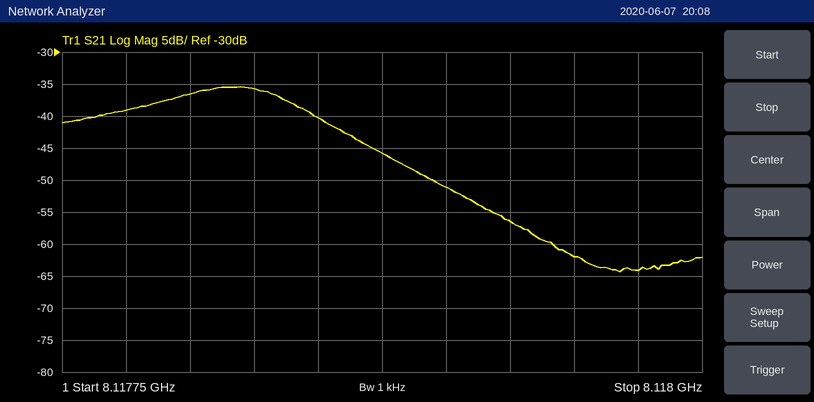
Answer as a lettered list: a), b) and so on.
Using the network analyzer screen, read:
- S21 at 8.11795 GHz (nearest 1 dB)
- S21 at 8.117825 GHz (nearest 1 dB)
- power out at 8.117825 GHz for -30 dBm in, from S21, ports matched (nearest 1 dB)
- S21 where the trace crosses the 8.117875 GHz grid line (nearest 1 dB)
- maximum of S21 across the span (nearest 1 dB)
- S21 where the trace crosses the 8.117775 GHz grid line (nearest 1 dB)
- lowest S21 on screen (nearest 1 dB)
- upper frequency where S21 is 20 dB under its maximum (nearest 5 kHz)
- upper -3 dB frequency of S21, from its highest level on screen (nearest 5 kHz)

a) -62 dB
b) -36 dB
c) -66 dBm
d) -46 dB
e) -35 dB
f) -39 dB
g) -64 dB
h) 8.117920 GHz
i) 8.117840 GHz
